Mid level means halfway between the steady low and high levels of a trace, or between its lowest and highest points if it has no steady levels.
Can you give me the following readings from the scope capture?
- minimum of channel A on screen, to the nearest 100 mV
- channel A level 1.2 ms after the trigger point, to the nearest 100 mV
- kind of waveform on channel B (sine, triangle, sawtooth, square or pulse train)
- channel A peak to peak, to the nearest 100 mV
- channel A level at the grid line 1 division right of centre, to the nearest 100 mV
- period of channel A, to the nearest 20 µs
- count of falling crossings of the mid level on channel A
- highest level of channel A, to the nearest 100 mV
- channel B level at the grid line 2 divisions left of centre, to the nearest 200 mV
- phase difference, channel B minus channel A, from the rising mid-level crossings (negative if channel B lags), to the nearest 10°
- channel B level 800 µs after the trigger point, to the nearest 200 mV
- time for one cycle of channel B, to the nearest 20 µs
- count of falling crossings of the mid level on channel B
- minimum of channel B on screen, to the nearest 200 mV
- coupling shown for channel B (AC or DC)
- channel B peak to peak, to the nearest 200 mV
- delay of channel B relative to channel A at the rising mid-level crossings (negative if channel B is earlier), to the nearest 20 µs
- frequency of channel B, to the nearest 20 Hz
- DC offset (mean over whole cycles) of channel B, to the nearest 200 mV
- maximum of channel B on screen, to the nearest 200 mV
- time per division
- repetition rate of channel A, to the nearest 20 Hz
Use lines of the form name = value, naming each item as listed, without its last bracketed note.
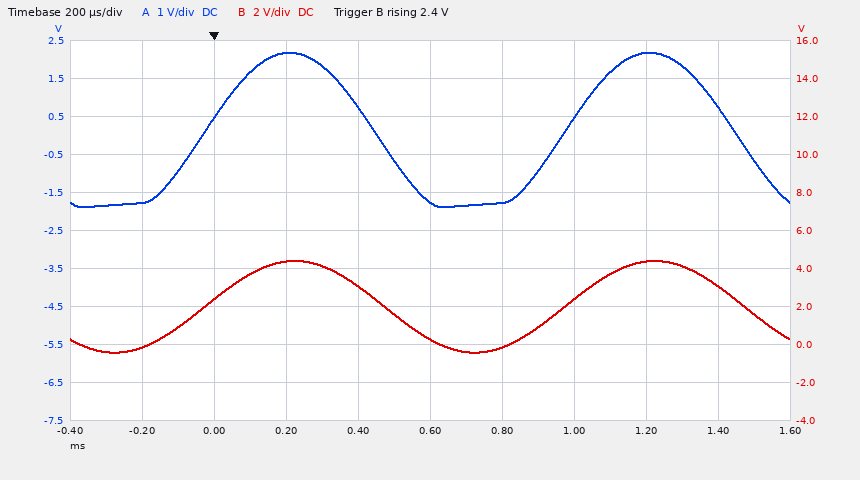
minimum of channel A on screen, to the nearest 100 mV = -1.9 V
channel A level 1.2 ms after the trigger point, to the nearest 100 mV = 2.2 V
kind of waveform on channel B = sine
channel A peak to peak, to the nearest 100 mV = 4.1 V
channel A level at the grid line 1 division right of centre, to the nearest 100 mV = -1.8 V
period of channel A, to the nearest 20 µs = 1.00 ms
count of falling crossings of the mid level on channel A = 2
highest level of channel A, to the nearest 100 mV = 2.2 V
channel B level at the grid line 2 divisions left of centre, to the nearest 200 mV = 4.4 V
phase difference, channel B minus channel A, from the rising mid-level crossings (negative if channel B lags), to the nearest 10° = 0°
channel B level 800 µs after the trigger point, to the nearest 200 mV = -200 mV
time for one cycle of channel B, to the nearest 20 µs = 1.00 ms
count of falling crossings of the mid level on channel B = 2
minimum of channel B on screen, to the nearest 200 mV = -400 mV
coupling shown for channel B = DC
channel B peak to peak, to the nearest 200 mV = 4.8 V
delay of channel B relative to channel A at the rising mid-level crossings (negative if channel B is earlier), to the nearest 20 µs = 0 µs
frequency of channel B, to the nearest 20 Hz = 1.00 kHz
DC offset (mean over whole cycles) of channel B, to the nearest 200 mV = 2.0 V
maximum of channel B on screen, to the nearest 200 mV = 4.4 V
time per division = 200 µs
repetition rate of channel A, to the nearest 20 Hz = 1.00 kHz
